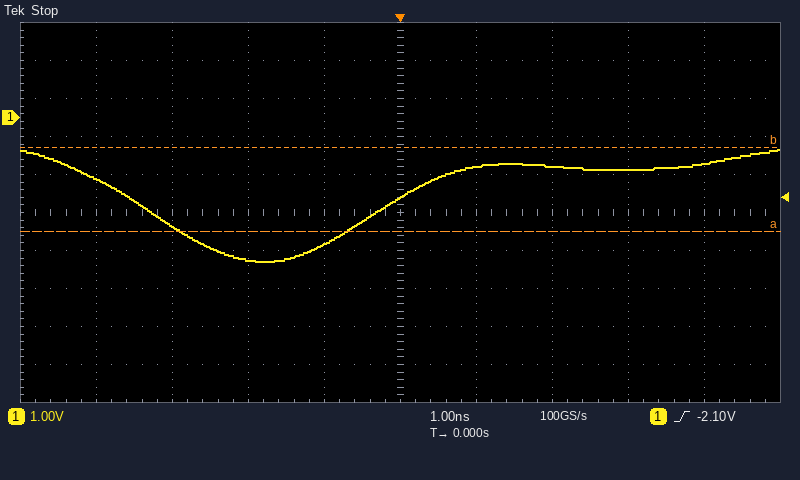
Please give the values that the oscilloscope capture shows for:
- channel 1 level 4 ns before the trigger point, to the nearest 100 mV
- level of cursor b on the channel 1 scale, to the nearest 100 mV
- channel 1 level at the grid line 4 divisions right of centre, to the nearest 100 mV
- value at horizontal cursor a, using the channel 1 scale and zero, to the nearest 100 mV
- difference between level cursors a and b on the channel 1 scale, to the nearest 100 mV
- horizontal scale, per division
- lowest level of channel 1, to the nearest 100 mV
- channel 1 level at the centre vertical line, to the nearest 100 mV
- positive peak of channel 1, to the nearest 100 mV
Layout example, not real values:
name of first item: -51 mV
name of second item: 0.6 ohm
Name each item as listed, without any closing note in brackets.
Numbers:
channel 1 level 4 ns before the trigger point, to the nearest 100 mV: -1.6 V
level of cursor b on the channel 1 scale, to the nearest 100 mV: -800 mV
channel 1 level at the grid line 4 divisions right of centre, to the nearest 100 mV: -1.2 V
value at horizontal cursor a, using the channel 1 scale and zero, to the nearest 100 mV: -3.0 V
difference between level cursors a and b on the channel 1 scale, to the nearest 100 mV: 2.2 V
horizontal scale, per division: 1 ns
lowest level of channel 1, to the nearest 100 mV: -3.8 V
channel 1 level at the centre vertical line, to the nearest 100 mV: -2.1 V
positive peak of channel 1, to the nearest 100 mV: -800 mV
